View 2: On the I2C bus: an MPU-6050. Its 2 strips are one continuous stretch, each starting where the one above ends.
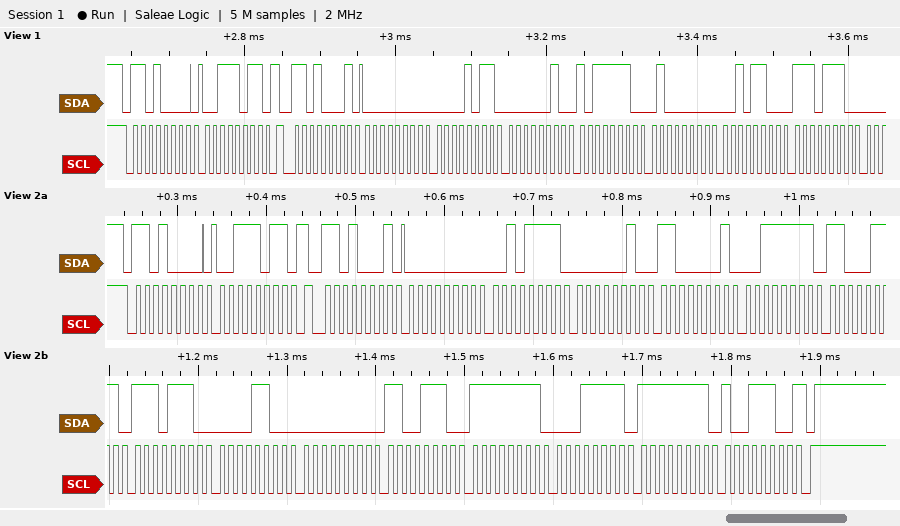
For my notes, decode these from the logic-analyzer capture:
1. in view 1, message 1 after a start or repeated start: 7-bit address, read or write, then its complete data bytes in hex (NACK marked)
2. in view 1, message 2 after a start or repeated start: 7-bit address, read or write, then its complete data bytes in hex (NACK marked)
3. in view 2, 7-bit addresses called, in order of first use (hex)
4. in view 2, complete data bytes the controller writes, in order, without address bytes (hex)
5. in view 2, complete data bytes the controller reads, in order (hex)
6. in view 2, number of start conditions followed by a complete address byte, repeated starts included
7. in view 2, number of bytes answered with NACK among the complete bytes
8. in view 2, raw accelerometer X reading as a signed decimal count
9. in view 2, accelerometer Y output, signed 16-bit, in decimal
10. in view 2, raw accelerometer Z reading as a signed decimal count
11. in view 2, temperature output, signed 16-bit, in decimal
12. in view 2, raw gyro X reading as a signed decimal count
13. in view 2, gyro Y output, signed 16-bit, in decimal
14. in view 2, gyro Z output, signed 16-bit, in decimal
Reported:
0x68 write: 3B
0x68 read: 00 0B 02 BE 40 2C EE
0x68
3B
00 2F 02 C1 3F C7 EE 0C 00 CE FF 1F FF 9C
2
1
47
705
16327
-4596
206
-225
-100
